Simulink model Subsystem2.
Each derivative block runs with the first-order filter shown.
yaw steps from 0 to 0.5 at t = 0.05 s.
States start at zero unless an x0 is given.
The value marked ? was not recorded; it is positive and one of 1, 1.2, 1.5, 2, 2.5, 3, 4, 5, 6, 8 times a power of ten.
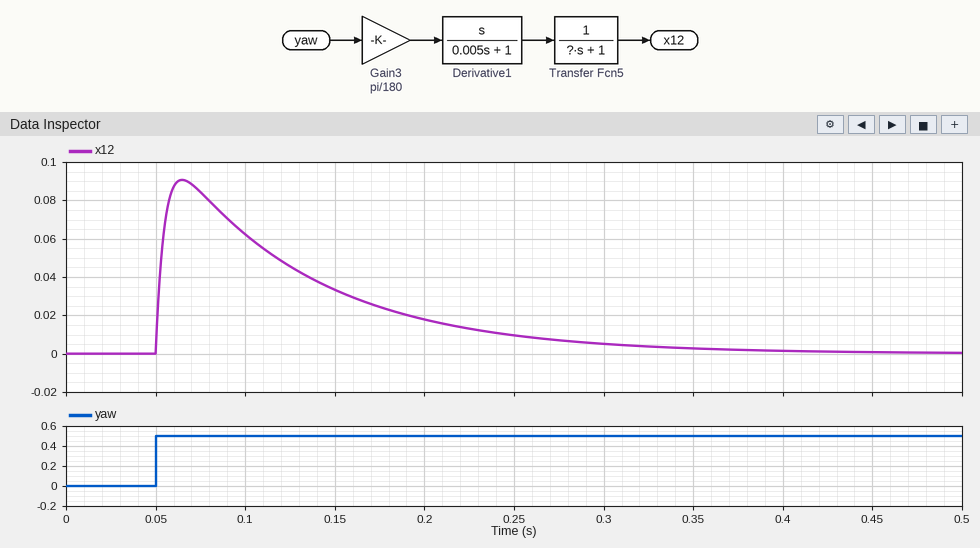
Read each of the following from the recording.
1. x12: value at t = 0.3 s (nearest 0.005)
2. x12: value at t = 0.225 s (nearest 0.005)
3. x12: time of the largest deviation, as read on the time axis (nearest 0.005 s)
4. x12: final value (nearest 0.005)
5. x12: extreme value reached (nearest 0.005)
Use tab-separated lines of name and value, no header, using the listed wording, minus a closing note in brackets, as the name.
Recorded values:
x12: value at t = 0.3 s	0.005
x12: value at t = 0.225 s	0.015
x12: time of the largest deviation, as read on the time axis	0.065 s
x12: final value	0.000
x12: extreme value reached	0.090
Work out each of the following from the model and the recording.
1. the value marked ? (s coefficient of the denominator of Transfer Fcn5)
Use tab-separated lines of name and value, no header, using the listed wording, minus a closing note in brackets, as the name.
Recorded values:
the value marked ?	0.08
